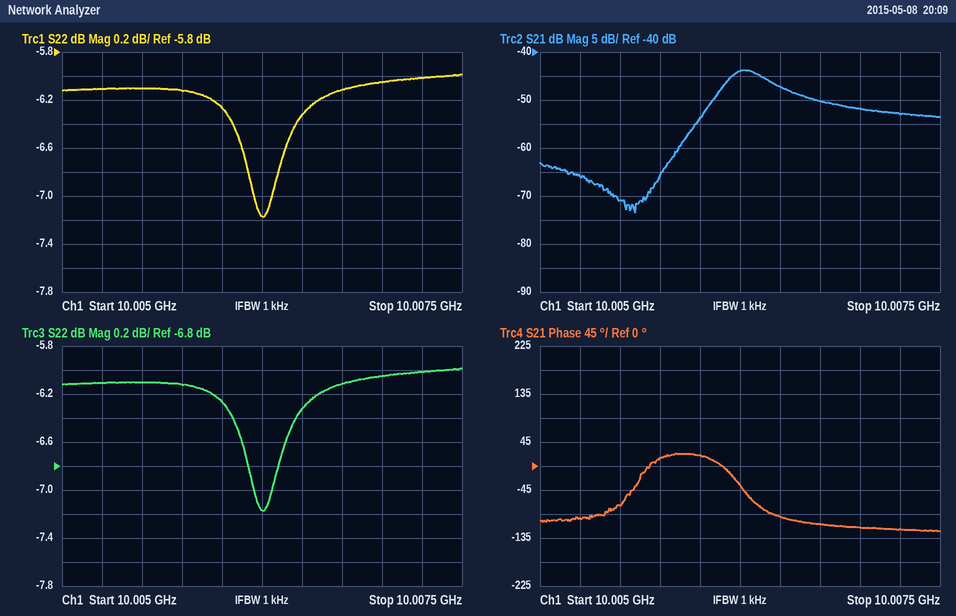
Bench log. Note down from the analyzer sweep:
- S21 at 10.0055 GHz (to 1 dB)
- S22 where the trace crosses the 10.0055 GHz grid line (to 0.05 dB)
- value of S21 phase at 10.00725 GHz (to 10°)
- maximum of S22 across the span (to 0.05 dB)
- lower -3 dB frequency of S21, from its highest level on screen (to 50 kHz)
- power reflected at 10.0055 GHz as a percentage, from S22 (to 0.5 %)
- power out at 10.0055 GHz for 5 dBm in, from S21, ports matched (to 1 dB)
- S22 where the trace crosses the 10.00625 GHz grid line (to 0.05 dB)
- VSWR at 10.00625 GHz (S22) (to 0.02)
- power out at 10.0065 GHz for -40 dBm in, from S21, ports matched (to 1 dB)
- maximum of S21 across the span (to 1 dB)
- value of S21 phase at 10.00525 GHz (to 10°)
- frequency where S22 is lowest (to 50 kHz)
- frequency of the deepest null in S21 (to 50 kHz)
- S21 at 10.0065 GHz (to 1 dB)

-71 dB
-6.10 dB
-120°
-6.00 dB
10.00615 GHz
24.5 %
-66 dBm
-7.15 dB
2.56
-87 dBm
-44 dB
-100°
10.00625 GHz
10.00560 GHz
-47 dB
